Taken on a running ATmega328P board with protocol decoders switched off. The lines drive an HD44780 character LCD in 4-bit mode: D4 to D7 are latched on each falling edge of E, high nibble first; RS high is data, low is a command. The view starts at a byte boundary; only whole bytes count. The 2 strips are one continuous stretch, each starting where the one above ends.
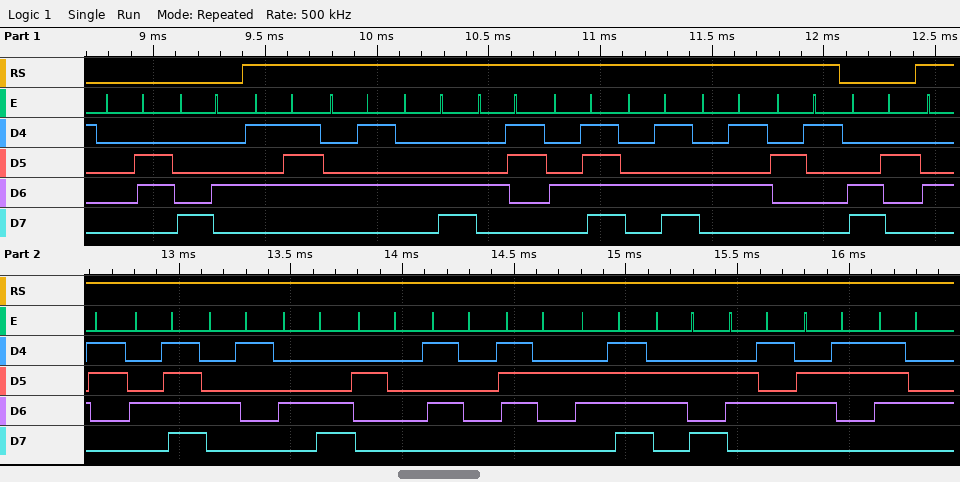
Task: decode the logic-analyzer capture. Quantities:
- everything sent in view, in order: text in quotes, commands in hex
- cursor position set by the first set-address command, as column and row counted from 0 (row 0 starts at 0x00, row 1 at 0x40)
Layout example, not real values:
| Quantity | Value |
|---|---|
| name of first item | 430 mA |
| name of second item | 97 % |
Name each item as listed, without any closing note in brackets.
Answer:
| Quantity | Value |
|---|---|
| everything sent in view, in order: text in quotes, commands in hex | 0x06 0x84 "WELCOME!" 0xC2 "COAL Project" |
| cursor position set by the first set-address command, as column and row counted from 0 | column 4, row 0 |
